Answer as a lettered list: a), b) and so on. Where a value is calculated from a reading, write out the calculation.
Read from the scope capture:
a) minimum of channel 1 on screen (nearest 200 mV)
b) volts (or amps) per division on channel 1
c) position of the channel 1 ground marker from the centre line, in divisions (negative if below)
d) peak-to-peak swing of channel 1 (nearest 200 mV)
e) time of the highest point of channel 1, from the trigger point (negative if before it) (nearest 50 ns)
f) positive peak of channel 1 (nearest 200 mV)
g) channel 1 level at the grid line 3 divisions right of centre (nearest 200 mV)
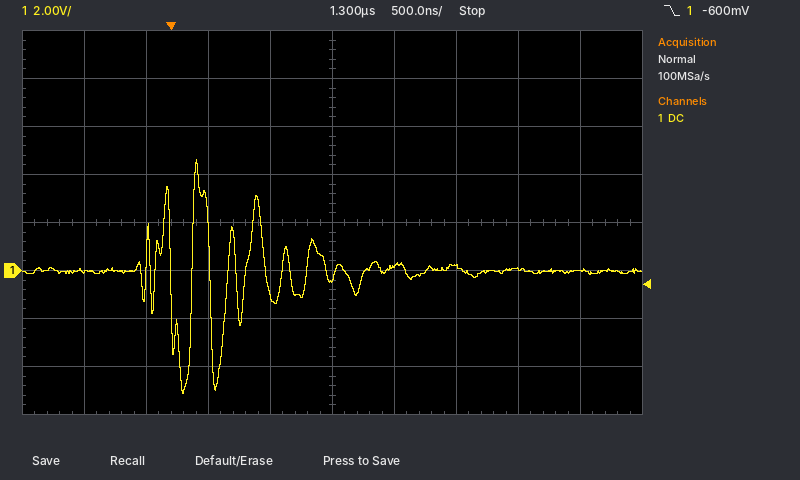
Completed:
a) -5.2 V
b) 2 V
c) -1.0 div
d) 4.6 V − (-5.2 V) = 9.8 V
e) +200 ns
f) 4.6 V
g) 0.0 V
